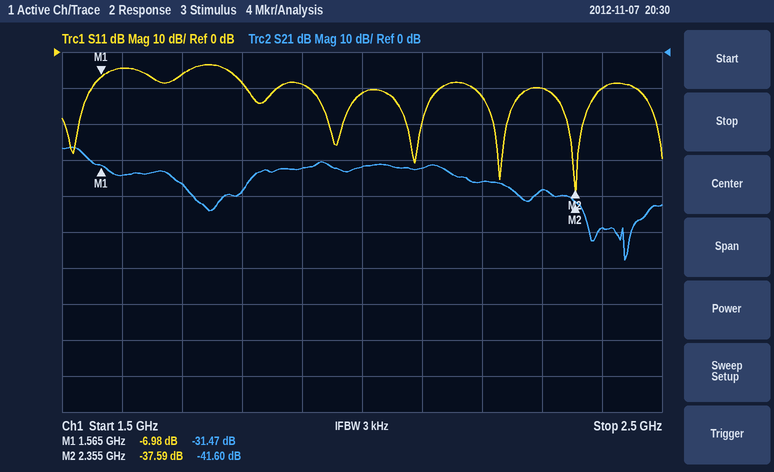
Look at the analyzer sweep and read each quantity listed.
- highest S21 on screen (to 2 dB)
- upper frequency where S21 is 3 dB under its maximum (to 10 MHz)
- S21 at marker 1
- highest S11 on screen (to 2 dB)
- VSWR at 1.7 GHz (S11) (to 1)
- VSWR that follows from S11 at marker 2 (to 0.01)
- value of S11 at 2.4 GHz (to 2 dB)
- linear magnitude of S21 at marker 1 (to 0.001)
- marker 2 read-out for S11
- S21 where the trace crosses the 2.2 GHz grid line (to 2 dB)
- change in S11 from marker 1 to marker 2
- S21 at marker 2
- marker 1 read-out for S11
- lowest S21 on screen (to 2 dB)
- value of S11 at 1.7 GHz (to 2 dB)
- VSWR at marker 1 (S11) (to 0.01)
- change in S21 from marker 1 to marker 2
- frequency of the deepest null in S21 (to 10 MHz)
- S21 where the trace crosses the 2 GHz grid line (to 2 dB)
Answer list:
-26 dB
1.54 GHz
-31.47 dB
-4 dB
3
1.03
-10 dB
0.027
-37.59 dB
-36 dB
-30.61 dB
-41.60 dB
-6.98 dB
-58 dB
-6 dB
2.62
-10.13 dB
2.44 GHz
-32 dB
